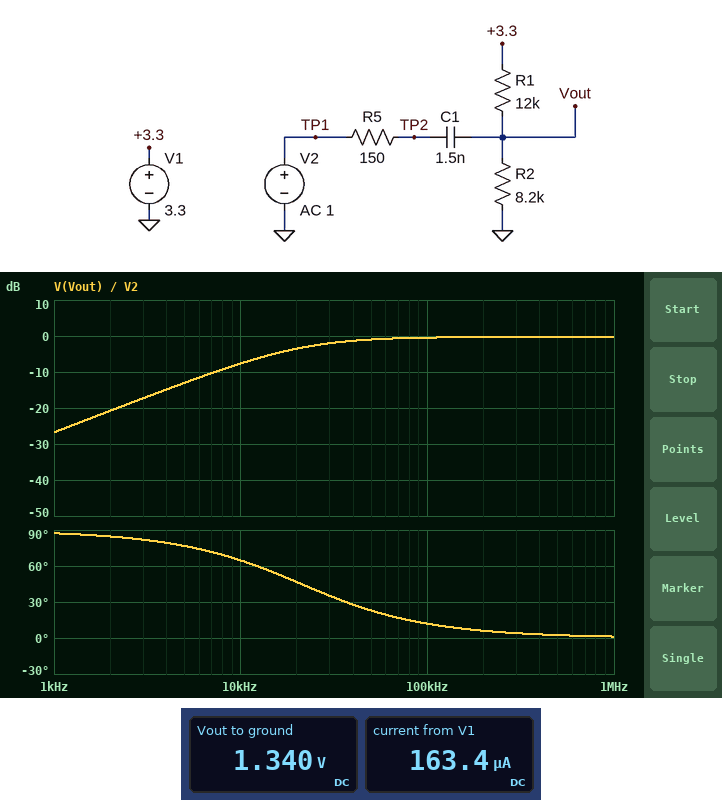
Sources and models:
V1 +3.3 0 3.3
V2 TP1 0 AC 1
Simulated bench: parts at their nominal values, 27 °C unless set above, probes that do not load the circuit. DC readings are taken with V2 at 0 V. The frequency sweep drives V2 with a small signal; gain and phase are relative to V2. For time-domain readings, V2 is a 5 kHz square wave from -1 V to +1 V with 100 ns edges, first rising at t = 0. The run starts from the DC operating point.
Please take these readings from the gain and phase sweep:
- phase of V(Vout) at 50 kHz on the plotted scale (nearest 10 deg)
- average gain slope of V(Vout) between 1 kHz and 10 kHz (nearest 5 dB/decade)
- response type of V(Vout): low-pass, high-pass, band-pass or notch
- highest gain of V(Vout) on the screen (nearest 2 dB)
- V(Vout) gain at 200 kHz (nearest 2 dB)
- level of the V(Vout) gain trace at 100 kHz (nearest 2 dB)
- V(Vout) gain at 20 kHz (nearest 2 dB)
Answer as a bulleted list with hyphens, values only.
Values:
- 20 deg
- 20 dB/decade
- high-pass
- 0 dB
- 0 dB
- 0 dB
- -4 dB
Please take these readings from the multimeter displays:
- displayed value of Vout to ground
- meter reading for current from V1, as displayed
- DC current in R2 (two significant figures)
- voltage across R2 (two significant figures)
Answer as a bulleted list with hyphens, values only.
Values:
- 1.340 V
- 163.4 µA
- 160 µA
- 1.3 V
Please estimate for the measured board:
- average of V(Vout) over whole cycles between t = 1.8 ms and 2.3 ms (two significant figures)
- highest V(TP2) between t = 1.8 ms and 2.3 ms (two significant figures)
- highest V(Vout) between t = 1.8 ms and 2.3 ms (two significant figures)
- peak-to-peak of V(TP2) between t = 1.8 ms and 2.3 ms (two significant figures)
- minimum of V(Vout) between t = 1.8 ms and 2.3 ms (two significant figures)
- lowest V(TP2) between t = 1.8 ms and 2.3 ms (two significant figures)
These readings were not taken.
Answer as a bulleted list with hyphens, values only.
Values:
- 1.3 V
- 1.0 V
- 3.3 V
- 2.0 V
- -590 mV
- -1.0 V
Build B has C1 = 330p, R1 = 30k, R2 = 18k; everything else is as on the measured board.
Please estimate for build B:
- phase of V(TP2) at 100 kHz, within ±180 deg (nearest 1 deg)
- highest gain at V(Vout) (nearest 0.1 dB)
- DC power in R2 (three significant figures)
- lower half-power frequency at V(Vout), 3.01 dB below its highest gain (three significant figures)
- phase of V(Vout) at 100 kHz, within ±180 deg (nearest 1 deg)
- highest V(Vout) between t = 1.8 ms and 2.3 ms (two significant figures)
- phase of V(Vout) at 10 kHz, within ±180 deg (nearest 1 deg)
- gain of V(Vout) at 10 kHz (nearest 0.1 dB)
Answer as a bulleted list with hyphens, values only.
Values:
- 0 deg
- -0.1 dB
- 85.1 µW
- 42.3 kHz
- 23 deg
- 3.2 V
- 77 deg
- -12.9 dB
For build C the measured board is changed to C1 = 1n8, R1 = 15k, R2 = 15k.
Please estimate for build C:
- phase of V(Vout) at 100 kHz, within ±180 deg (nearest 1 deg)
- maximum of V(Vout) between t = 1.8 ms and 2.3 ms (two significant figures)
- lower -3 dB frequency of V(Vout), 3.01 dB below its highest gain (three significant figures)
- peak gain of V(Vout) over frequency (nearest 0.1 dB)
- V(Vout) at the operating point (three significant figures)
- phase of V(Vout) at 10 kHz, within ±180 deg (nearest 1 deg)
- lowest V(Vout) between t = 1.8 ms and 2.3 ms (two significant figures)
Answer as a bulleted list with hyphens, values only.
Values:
- 7 deg
- 3.6 V
- 11.6 kHz
- -0.2 dB
- 1.65 V
- 49 deg
- -300 mV
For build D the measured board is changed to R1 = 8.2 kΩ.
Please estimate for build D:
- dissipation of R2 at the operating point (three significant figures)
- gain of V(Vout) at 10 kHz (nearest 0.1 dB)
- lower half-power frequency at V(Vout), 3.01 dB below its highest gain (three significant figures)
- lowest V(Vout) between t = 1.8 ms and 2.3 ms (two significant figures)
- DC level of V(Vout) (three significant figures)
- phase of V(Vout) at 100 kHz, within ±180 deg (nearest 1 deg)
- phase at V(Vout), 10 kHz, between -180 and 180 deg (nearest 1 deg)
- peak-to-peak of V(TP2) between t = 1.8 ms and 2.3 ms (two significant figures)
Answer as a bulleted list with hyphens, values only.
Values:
- 332 µW
- -8.9 dB
- 25.0 kHz
- -260 mV
- 1.65 V
- 14 deg
- 68 deg
- 2.0 V
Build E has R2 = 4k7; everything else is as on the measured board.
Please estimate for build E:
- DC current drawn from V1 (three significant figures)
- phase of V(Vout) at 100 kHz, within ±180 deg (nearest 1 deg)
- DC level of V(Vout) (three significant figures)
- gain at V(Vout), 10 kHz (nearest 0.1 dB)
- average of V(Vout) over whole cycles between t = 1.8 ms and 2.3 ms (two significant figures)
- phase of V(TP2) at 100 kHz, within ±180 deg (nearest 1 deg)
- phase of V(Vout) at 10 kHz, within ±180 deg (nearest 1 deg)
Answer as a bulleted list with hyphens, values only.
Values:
- 198 µA
- 17 deg
- 929 mV
- -10.4 dB
- 930 mV
- -1 deg
- 72 deg
